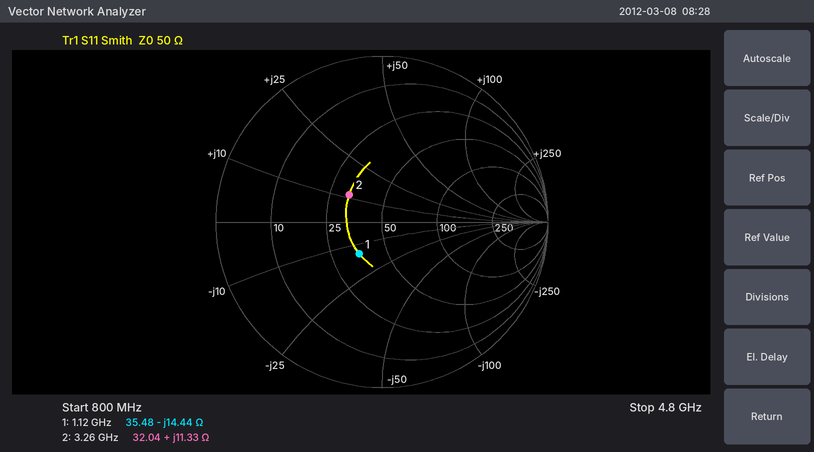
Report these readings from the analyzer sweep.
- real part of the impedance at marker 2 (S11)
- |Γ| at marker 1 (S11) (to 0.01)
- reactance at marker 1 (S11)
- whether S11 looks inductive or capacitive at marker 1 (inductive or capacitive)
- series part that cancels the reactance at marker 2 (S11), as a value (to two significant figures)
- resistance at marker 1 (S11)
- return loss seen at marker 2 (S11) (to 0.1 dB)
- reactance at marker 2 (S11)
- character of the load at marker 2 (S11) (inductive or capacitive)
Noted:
32.04 Ω
0.24
-14.44 Ω
capacitive
4.3 pF
35.48 Ω
11.8 dB
+11.33 Ω
inductive
